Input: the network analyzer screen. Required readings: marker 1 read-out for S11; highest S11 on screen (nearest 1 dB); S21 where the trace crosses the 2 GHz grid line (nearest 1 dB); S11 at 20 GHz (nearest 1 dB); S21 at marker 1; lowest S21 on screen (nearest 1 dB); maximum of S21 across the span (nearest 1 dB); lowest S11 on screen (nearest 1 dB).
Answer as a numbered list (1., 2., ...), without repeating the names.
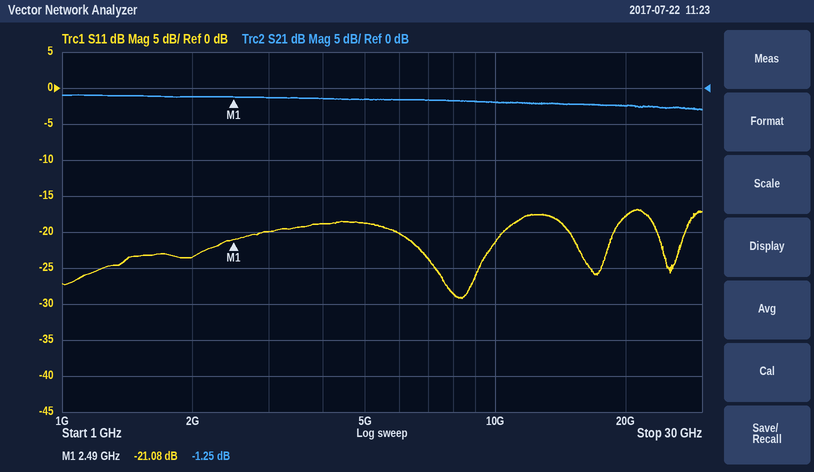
1. -21.08 dB
2. -17 dB
3. -1 dB
4. -18 dB
5. -1.25 dB
6. -3 dB
7. -1 dB
8. -29 dB
